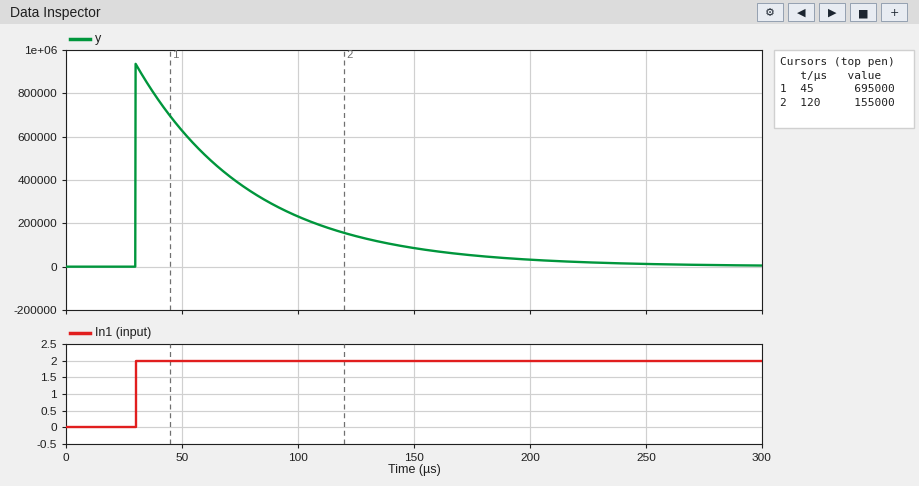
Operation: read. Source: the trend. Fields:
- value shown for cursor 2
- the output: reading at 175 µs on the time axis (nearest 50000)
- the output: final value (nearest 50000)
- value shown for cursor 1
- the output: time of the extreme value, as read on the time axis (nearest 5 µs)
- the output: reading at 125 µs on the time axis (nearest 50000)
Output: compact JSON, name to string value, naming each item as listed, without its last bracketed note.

{"value shown for cursor 2": "155000", "the output: reading at 175 µs on the time axis": "50000", "the output: final value": "0", "value shown for cursor 1": "695000", "the output: time of the extreme value, as read on the time axis": "30 µs", "the output: reading at 125 µs on the time axis": "150000"}
